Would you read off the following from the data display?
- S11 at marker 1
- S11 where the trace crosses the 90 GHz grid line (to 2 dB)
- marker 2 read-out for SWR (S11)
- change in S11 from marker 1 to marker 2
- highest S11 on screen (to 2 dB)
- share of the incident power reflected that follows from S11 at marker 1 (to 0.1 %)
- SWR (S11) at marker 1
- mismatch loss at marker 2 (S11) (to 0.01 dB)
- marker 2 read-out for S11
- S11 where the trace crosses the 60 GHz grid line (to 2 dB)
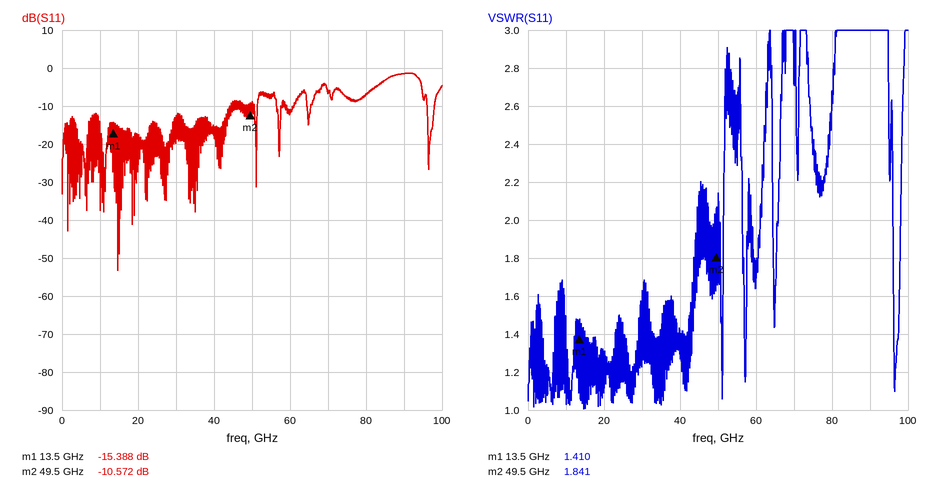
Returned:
-15.388 dB
-2 dB
1.841
4.816 dB
-2 dB
2.9 %
1.410
0.40 dB
-10.572 dB
-12 dB
